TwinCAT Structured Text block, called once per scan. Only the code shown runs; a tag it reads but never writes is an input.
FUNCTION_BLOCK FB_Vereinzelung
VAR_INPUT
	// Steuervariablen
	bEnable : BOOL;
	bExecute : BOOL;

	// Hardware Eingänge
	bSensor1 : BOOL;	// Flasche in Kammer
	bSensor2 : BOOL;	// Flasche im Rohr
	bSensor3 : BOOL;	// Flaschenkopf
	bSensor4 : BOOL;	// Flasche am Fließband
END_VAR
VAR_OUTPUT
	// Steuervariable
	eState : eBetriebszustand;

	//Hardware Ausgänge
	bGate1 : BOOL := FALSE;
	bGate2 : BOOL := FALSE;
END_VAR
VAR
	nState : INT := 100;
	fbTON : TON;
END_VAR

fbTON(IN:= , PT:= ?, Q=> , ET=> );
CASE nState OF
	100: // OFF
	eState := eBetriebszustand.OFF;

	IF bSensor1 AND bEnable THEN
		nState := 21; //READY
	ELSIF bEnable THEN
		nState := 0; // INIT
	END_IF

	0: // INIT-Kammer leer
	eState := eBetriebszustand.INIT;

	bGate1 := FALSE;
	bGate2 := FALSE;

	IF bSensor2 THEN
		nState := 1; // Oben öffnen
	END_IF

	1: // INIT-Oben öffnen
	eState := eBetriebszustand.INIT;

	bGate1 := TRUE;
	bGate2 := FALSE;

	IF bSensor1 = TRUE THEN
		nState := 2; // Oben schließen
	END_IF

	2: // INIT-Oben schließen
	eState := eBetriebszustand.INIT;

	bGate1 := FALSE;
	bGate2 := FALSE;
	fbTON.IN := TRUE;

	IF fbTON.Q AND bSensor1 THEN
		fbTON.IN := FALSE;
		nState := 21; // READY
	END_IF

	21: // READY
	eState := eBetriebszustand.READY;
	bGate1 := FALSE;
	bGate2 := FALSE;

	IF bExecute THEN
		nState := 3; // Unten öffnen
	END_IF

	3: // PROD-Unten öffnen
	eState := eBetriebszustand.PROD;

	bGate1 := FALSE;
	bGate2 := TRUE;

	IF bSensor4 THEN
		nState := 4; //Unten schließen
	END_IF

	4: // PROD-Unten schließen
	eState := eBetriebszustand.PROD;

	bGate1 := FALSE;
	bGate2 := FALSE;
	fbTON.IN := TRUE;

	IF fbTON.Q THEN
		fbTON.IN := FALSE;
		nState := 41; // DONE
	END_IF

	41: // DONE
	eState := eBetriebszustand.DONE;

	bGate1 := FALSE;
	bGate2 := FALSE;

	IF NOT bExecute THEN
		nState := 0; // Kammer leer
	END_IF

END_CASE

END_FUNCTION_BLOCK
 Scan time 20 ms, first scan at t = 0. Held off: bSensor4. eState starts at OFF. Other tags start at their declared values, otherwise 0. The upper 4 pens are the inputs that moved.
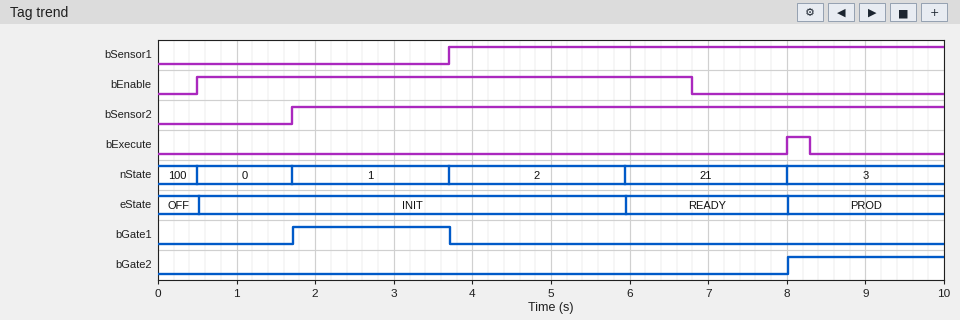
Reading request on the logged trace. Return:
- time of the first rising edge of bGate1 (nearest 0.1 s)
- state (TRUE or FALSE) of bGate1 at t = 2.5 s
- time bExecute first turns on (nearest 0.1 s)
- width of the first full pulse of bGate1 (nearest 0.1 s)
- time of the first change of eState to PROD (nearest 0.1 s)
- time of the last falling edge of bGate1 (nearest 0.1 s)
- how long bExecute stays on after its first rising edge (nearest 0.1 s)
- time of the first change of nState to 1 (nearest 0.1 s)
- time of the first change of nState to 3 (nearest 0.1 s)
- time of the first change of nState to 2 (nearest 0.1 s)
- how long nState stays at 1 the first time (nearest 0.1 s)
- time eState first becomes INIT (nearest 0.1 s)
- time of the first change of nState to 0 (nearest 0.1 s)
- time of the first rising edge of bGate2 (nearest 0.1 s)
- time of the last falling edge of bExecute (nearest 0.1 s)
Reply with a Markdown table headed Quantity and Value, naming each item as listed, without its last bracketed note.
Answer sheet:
| Quantity | Value |
|---|---|
| time of the first rising edge of bGate1 | 1.7 s |
| state (TRUE or FALSE) of bGate1 at t = 2.5 s | TRUE |
| time bExecute first turns on | 8.0 s |
| width of the first full pulse of bGate1 | 2.0 s |
| time of the first change of eState to PROD | 8.0 s |
| time of the last falling edge of bGate1 | 3.7 s |
| how long bExecute stays on after its first rising edge | 0.3 s |
| time of the first change of nState to 1 | 1.7 s |
| time of the first change of nState to 3 | 8.0 s |
| time of the first change of nState to 2 | 3.7 s |
| how long nState stays at 1 the first time | 2.0 s |
| time eState first becomes INIT | 0.5 s |
| time of the first change of nState to 0 | 0.5 s |
| time of the first rising edge of bGate2 | 8.0 s |
| time of the last falling edge of bExecute | 8.3 s |
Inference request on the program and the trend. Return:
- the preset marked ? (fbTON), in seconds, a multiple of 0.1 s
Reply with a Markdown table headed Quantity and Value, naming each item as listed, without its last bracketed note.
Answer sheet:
| Quantity | Value |
|---|---|
| the preset marked ? (fbTON), in seconds, a multiple of 0.1 s | 2.2 s |
